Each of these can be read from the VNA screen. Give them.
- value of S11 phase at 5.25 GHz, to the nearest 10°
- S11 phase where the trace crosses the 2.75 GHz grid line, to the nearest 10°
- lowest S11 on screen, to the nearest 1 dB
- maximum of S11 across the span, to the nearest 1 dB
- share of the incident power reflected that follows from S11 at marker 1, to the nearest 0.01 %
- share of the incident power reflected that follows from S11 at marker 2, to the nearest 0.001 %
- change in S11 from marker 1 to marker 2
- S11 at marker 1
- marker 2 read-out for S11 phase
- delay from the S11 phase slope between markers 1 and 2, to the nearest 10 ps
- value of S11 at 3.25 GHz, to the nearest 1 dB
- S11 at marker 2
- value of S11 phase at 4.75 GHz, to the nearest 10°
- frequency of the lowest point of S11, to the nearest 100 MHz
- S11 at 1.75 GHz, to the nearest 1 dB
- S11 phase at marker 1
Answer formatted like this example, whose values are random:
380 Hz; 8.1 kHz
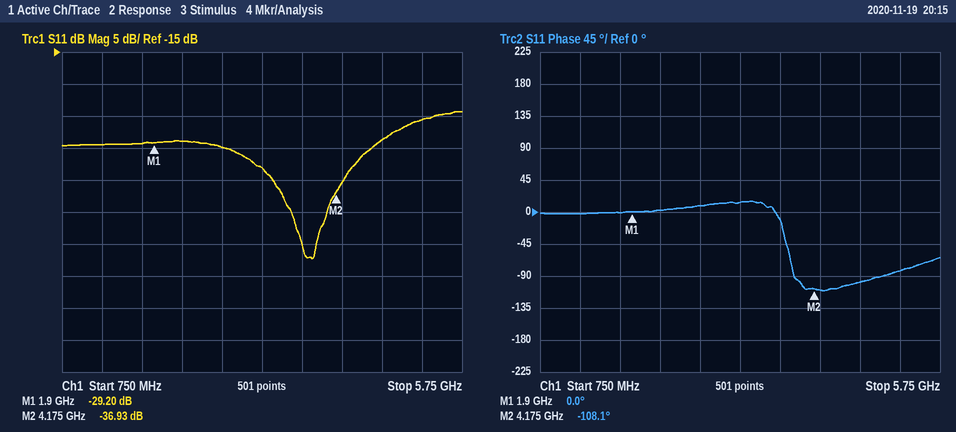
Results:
-80°; 10°; -47 dB; -24 dB; 0.12 %; 0.020 %; -7.73 dB; -29.20 dB; -108.1°; 130 ps; -33 dB; -36.93 dB; -100°; 3.9 GHz; -29 dB; 0.0°
